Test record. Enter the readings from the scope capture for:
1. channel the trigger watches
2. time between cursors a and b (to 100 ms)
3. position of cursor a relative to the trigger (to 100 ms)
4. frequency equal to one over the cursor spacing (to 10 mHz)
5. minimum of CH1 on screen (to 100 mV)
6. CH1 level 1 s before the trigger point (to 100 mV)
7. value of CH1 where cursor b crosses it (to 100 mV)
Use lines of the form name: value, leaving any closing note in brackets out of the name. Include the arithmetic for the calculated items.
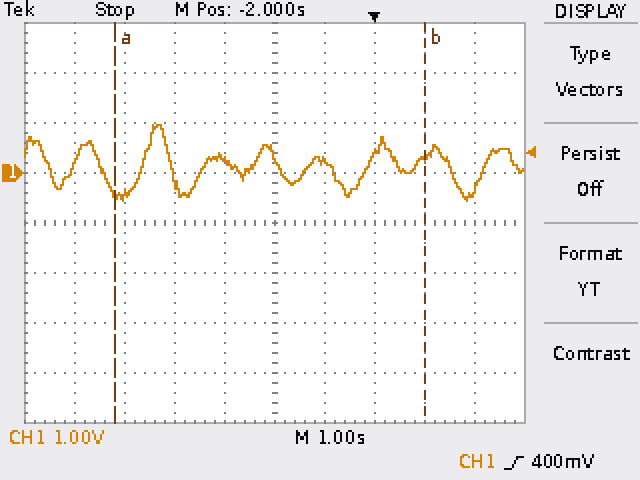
channel the trigger watches: CH1
time between cursors a and b: 6.2 s
position of cursor a relative to the trigger: -5.2 s
frequency equal to one over the cursor spacing: 1 / 6.2 s ≈ 160 mHz
minimum of CH1 on screen: -600 mV
CH1 level 1 s before the trigger point: 200 mV
value of CH1 where cursor b crosses it: 300 mV
